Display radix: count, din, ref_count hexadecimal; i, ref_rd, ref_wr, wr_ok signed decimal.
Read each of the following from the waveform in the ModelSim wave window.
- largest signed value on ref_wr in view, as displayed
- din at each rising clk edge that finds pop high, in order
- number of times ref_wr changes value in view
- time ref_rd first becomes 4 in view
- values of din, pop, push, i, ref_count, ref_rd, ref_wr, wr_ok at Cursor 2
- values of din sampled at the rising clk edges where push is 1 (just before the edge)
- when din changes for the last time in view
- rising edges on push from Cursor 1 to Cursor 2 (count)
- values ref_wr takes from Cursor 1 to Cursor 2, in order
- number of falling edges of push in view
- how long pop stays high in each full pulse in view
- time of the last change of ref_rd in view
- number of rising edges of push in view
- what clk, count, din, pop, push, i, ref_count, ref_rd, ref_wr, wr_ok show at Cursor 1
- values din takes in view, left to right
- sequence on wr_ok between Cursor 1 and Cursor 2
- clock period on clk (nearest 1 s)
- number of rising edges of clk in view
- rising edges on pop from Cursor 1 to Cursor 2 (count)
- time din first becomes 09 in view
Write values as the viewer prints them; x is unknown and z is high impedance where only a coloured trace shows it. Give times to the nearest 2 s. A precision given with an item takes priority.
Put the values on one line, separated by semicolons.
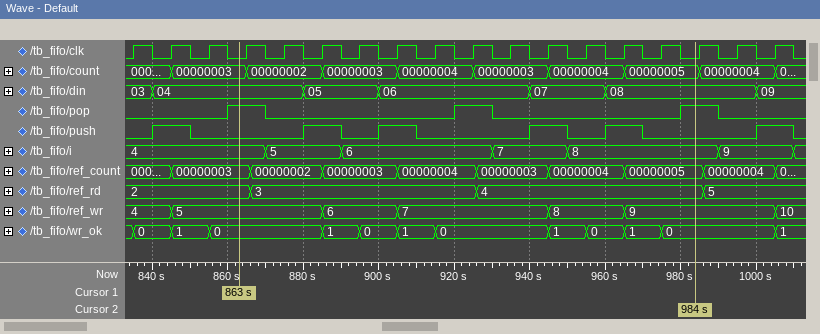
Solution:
10; 04, 06, 08; 6; 926 s; din=08, pop=1, push=0, i=8, ref_count=00000005, ref_rd=4, ref_wr=9, wr_ok=0; 04, 05, 06, 07, 08, 09; 1000 s; 4; 5, 6, 7, 8, 9; 6; 10 s, 10 s, 10 s; 986 s; 6; clk=0, count=00000003, din=04, pop=1, push=0, i=4, ref_count=00000003, ref_rd=2, ref_wr=5, wr_ok=0; 03, 04, 05, 06, 07, 08, 09; 0, 1, 0, 1, 0, 1, 0, 1, 0; 10 s; 18; 2; 1000 s
